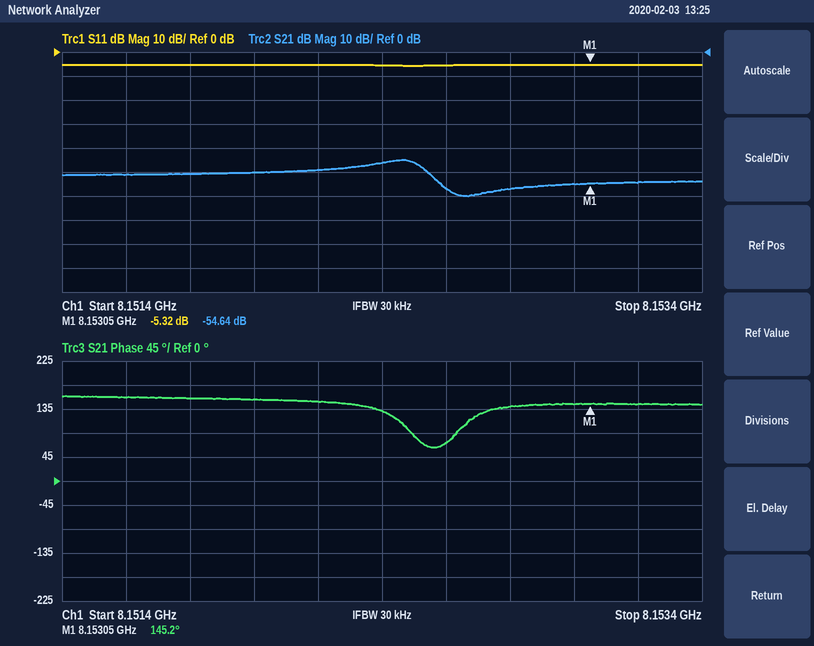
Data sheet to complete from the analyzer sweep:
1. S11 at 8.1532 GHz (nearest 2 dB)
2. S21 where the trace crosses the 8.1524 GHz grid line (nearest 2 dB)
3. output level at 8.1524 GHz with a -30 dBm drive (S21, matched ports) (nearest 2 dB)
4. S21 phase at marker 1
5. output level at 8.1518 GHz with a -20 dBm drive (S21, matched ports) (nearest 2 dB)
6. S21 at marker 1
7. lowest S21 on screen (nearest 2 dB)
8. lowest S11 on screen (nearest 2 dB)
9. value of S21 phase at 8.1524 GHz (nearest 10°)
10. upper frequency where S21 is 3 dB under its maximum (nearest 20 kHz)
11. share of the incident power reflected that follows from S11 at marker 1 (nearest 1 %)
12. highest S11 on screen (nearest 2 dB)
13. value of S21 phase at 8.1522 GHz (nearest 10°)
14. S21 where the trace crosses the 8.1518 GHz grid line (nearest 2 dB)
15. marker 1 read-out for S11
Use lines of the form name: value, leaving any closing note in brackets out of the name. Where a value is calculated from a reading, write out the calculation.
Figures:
S11 at 8.1532 GHz: -6 dB
S21 where the trace crosses the 8.1524 GHz grid line: -46 dB
output level at 8.1524 GHz with a -30 dBm drive (S21, matched ports): -30 dBm + (-46 dB) = -76 dBm
S21 phase at marker 1: 145.2°
output level at 8.1518 GHz with a -20 dBm drive (S21, matched ports): -20 dBm + (-50 dB) = -70 dBm
S21 at marker 1: -54.64 dB
lowest S21 on screen: -60 dB
lowest S11 on screen: -6 dB
value of S21 phase at 8.1524 GHz: 130°
upper frequency where S21 is 3 dB under its maximum: 8.15252 GHz
share of the incident power reflected that follows from S11 at marker 1: 10^(-5.32/10) ≈ 29 %
highest S11 on screen: -6 dB
value of S21 phase at 8.1522 GHz: 150°
S21 where the trace crosses the 8.1518 GHz grid line: -50 dB
marker 1 read-out for S11: -5.32 dB
